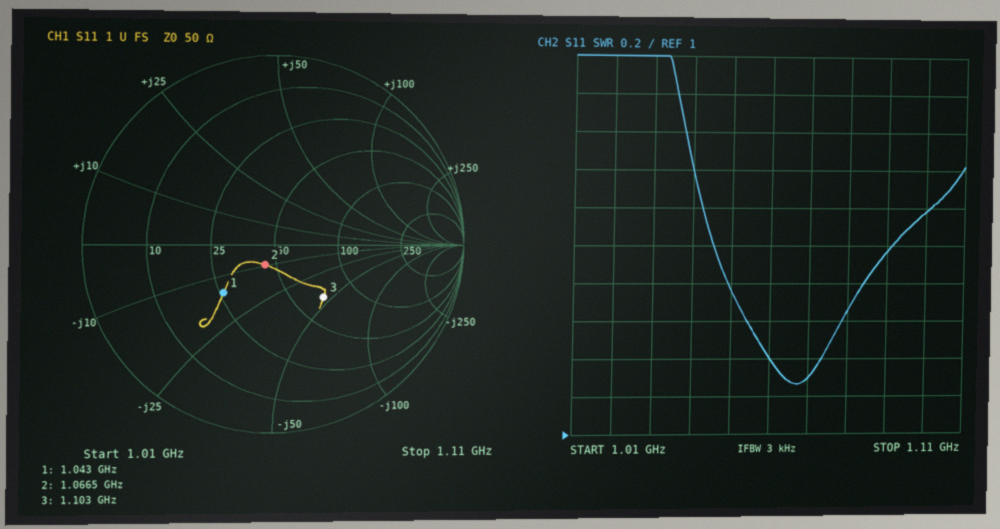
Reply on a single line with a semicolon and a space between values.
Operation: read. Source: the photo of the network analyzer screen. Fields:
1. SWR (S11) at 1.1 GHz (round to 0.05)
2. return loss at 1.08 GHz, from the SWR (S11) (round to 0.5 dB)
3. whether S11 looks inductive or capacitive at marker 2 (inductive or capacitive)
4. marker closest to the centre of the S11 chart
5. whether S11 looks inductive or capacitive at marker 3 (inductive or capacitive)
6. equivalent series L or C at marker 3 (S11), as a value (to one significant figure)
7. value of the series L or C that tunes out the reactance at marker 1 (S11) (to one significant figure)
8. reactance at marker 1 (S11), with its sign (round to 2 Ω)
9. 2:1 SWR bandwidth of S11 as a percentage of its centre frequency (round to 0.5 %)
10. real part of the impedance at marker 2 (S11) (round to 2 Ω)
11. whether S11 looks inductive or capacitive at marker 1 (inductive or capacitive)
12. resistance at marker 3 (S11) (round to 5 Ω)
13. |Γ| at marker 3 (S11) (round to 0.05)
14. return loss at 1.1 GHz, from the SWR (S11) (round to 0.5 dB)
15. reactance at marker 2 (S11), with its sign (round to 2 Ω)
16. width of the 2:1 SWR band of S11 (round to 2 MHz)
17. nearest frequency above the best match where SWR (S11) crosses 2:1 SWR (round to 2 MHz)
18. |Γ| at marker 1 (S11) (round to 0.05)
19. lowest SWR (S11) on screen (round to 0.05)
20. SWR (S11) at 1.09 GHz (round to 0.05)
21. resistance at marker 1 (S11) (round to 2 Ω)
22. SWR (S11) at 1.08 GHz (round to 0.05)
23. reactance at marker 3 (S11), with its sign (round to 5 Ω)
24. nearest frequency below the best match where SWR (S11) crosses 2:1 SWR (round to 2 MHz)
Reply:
2.20; 12.0 dB; capacitive; marker 2; capacitive; 3 pF; 2 nH; -16 Ω; 4.5 %; 44 Ω; capacitive; 70 Ω; 0.40; 8.5 dB; -10 Ω; 46 MHz; 1.092 GHz; 0.35; 1.25; 1.95; 26 Ω; 1.65; -45 Ω; 1.046 GHz
